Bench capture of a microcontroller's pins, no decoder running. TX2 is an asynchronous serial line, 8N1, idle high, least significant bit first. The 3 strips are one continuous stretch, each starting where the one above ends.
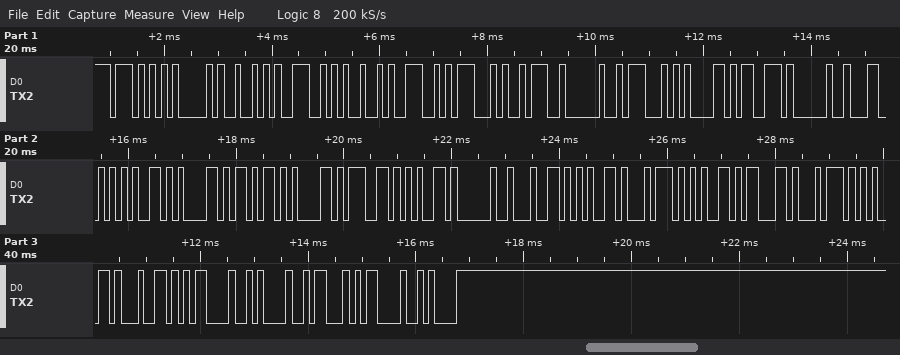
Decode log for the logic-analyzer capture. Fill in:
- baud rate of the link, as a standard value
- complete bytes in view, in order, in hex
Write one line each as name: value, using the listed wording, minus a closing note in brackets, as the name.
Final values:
baud rate of the link, as a standard value: 9600 baud
complete bytes in view, in order, in hex: 0x57 0x41 0x52 0x4E 0x49 0x4E 0x47 0x3A 0x20 0x47 0x61 0x73 0x20 0x4C 0x65 0x61 0x6B 0x61 0x67 0x65 0x20 0x64 0x65 0x74 0x65 0x63 0x74 0x65 0x64 0x0D 0x0A 0x1A 0x0D 0x0A
